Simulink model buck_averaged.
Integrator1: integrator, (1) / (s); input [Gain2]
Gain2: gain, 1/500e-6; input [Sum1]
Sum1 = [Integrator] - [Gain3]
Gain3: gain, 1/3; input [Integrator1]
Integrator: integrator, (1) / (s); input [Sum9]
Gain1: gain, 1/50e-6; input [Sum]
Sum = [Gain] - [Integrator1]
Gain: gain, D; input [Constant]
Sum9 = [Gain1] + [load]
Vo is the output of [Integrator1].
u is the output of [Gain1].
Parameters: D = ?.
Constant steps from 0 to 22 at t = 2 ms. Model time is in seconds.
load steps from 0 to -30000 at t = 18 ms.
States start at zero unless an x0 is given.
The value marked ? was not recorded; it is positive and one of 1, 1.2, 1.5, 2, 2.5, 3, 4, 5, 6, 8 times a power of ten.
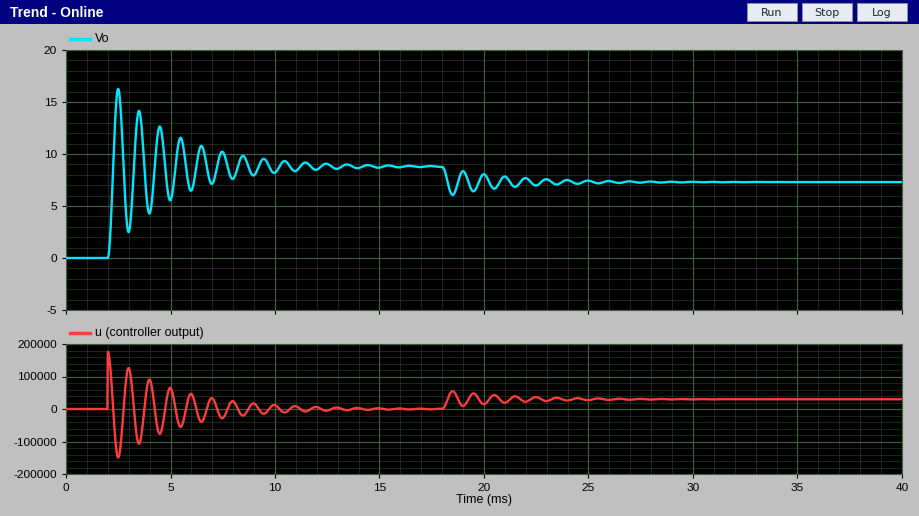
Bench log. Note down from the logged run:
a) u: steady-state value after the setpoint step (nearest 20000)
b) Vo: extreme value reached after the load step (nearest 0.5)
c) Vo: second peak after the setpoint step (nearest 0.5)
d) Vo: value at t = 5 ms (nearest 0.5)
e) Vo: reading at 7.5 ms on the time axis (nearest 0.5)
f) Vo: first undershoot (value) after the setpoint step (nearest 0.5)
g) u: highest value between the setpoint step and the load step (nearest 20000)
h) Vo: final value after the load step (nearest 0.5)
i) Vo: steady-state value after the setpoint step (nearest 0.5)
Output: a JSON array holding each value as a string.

["0", "6.0", "14.0", "5.5", "10.0", "2.5", "180000", "7.5", "9.0"]
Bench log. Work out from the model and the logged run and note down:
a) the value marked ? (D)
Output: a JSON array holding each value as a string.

["0.4"]
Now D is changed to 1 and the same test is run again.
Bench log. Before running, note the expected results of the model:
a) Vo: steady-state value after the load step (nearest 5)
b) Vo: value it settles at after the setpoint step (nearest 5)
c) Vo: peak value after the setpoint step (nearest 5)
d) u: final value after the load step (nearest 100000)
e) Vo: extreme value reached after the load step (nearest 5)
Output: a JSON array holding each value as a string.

["20", "20", "40", "0", "20"]
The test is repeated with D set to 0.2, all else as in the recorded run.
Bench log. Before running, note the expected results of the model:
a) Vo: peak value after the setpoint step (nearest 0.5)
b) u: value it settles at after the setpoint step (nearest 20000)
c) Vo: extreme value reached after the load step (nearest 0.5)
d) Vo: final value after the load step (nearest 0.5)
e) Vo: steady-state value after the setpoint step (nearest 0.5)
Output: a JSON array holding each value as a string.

["8.0", "0", "1.5", "3.0", "4.5"]
